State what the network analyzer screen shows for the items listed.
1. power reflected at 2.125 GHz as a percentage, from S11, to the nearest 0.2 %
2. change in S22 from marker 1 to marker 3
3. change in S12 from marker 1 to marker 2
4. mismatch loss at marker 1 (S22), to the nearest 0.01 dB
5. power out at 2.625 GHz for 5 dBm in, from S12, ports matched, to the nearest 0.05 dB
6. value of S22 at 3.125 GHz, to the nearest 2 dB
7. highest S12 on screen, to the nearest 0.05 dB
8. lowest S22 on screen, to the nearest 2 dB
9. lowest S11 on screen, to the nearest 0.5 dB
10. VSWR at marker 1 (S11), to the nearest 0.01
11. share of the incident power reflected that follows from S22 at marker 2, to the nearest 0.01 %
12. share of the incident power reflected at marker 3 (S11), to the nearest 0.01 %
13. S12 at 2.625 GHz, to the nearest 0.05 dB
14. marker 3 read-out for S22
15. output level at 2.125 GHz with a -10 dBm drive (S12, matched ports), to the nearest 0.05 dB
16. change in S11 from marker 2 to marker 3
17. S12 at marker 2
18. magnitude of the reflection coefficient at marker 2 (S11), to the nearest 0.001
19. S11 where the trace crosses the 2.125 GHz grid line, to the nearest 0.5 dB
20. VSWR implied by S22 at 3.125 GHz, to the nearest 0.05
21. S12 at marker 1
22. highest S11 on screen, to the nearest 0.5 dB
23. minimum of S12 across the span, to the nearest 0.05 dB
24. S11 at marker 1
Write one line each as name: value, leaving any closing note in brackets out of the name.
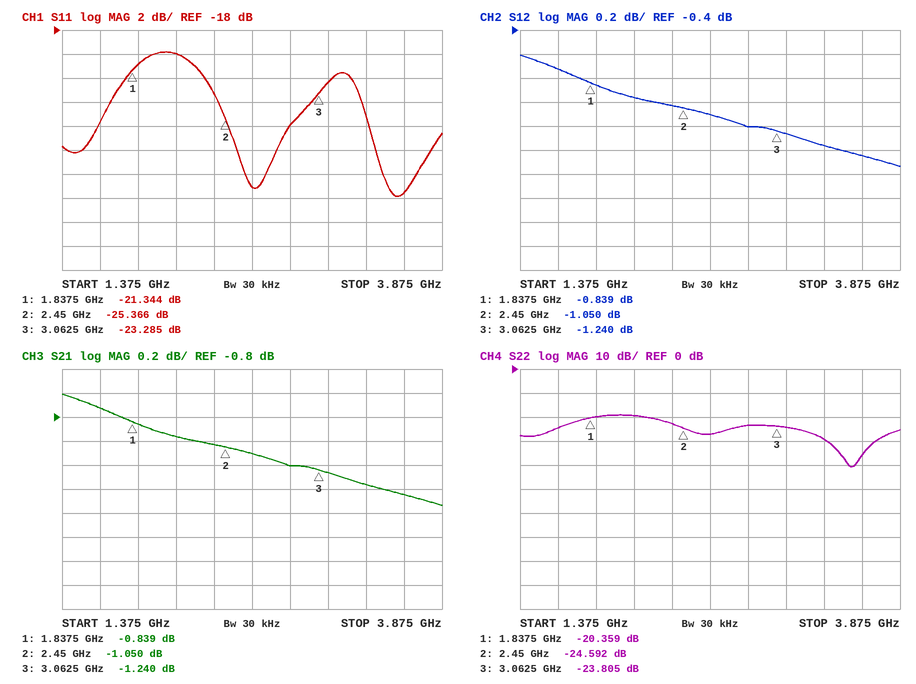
power reflected at 2.125 GHz as a percentage, from S11, to the nearest 0.2 %: 1.0 %
change in S22 from marker 1 to marker 3: -3.446 dB
change in S12 from marker 1 to marker 2: -0.211 dB
mismatch loss at marker 1 (S22), to the nearest 0.01 dB: 0.04 dB
power out at 2.625 GHz for 5 dBm in, from S12, ports matched, to the nearest 0.05 dB: 3.90 dBm
value of S22 at 3.125 GHz, to the nearest 2 dB: -24 dB
highest S12 on screen, to the nearest 0.05 dB: -0.60 dB
lowest S22 on screen, to the nearest 2 dB: -40 dB
lowest S11 on screen, to the nearest 0.5 dB: -32.0 dB
VSWR at marker 1 (S11), to the nearest 0.01: 1.19
share of the incident power reflected that follows from S22 at marker 2, to the nearest 0.01 %: 0.35 %
share of the incident power reflected at marker 3 (S11), to the nearest 0.01 %: 0.47 %
S12 at 2.625 GHz, to the nearest 0.05 dB: -1.10 dB
marker 3 read-out for S22: -23.805 dB
output level at 2.125 GHz with a -10 dBm drive (S12, matched ports), to the nearest 0.05 dB: -10.95 dBm
change in S11 from marker 2 to marker 3: 2.081 dB
S12 at marker 2: -1.050 dB
magnitude of the reflection coefficient at marker 2 (S11), to the nearest 0.001: 0.054
S11 where the trace crosses the 2.125 GHz grid line, to the nearest 0.5 dB: -20.0 dB
VSWR implied by S22 at 3.125 GHz, to the nearest 0.05: 1.15
S12 at marker 1: -0.839 dB
highest S11 on screen, to the nearest 0.5 dB: -20.0 dB
minimum of S12 across the span, to the nearest 0.05 dB: -1.55 dB
S11 at marker 1: -21.344 dB
